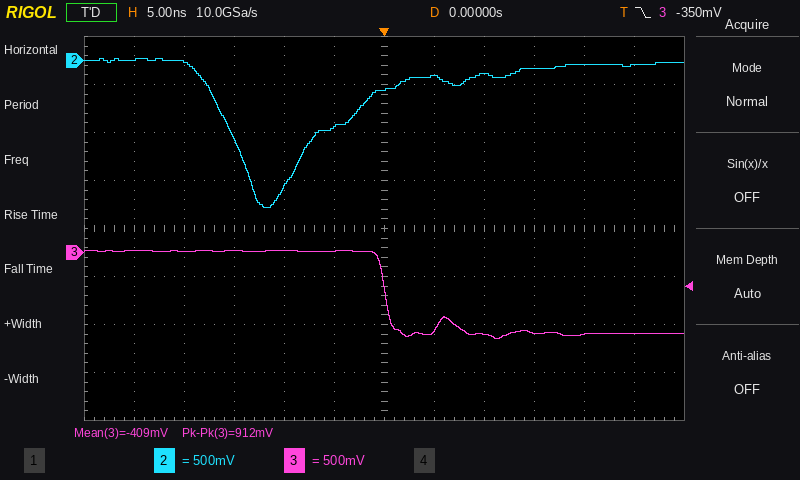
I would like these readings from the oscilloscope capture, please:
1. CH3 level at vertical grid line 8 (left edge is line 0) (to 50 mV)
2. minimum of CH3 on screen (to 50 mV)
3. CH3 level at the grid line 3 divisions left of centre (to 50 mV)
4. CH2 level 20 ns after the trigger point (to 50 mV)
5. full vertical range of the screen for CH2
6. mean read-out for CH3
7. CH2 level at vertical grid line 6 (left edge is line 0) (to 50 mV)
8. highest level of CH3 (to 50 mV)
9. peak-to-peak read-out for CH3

-850 mV
-900 mV
0 mV
-50 mV
4 V
-409 mV
-300 mV
0 mV
912 mV
